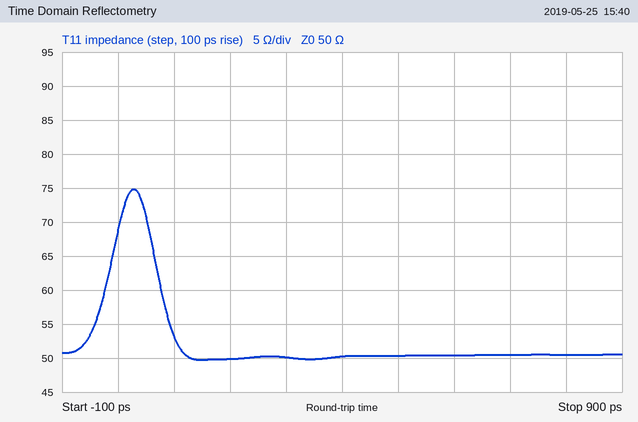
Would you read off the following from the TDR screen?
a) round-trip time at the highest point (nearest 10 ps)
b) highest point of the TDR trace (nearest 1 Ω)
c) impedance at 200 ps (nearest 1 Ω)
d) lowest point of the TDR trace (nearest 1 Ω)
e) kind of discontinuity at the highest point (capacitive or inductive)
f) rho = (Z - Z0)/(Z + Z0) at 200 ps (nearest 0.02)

30 ps
75 Ω
50 Ω
50 Ω
inductive
0.00
